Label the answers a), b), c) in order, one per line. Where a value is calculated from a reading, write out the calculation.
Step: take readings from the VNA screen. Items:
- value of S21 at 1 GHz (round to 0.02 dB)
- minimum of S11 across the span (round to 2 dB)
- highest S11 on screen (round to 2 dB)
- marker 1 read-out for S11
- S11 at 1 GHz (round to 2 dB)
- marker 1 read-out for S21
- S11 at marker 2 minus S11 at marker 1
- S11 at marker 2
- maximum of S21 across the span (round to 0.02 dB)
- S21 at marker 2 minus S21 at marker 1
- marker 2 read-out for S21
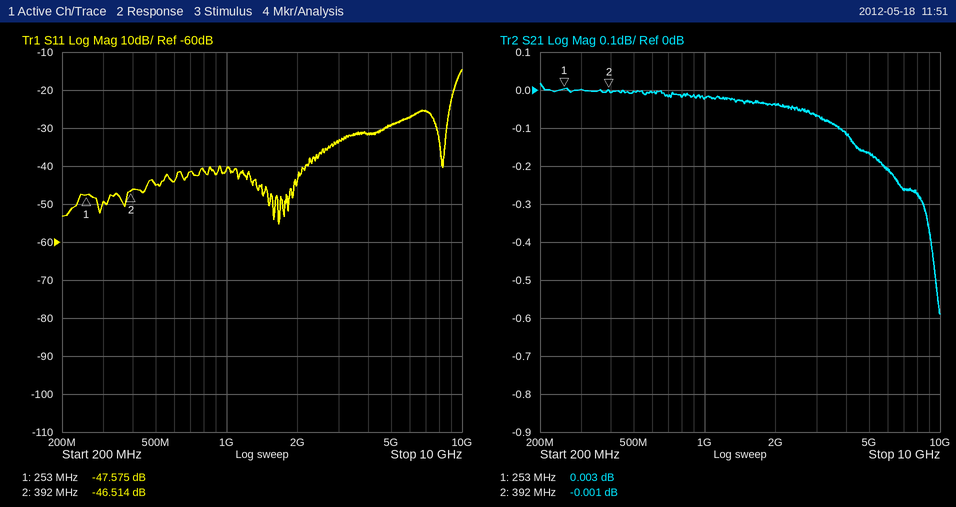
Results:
a) -0.02 dB
b) -56 dB
c) -14 dB
d) -47.575 dB
e) -40 dB
f) 0.003 dB
g) -46.514 − (-47.575) = 1.061 dB
h) -46.514 dB
i) 0.02 dB
j) -0.001 − (0.003) = -0.004 dB
k) -0.001 dB
